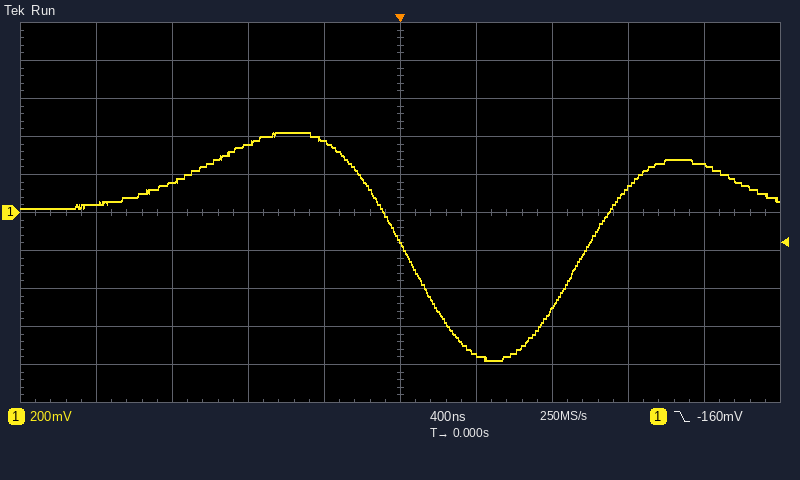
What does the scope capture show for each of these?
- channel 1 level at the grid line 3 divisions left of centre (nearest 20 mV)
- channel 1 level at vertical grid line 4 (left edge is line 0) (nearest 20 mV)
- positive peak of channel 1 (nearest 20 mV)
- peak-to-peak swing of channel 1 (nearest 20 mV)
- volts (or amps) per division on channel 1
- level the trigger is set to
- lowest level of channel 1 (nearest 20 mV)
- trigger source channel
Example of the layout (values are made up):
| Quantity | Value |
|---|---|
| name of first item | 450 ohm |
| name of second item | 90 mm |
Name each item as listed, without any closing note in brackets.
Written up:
| Quantity | Value |
|---|---|
| channel 1 level at the grid line 3 divisions left of centre | 160 mV |
| channel 1 level at vertical grid line 4 (left edge is line 0) | 380 mV |
| positive peak of channel 1 | 420 mV |
| peak-to-peak swing of channel 1 | 1.20 V |
| volts (or amps) per division on channel 1 | 200 mV |
| level the trigger is set to | -160 mV |
| lowest level of channel 1 | -780 mV |
| trigger source channel | channel 1 |
